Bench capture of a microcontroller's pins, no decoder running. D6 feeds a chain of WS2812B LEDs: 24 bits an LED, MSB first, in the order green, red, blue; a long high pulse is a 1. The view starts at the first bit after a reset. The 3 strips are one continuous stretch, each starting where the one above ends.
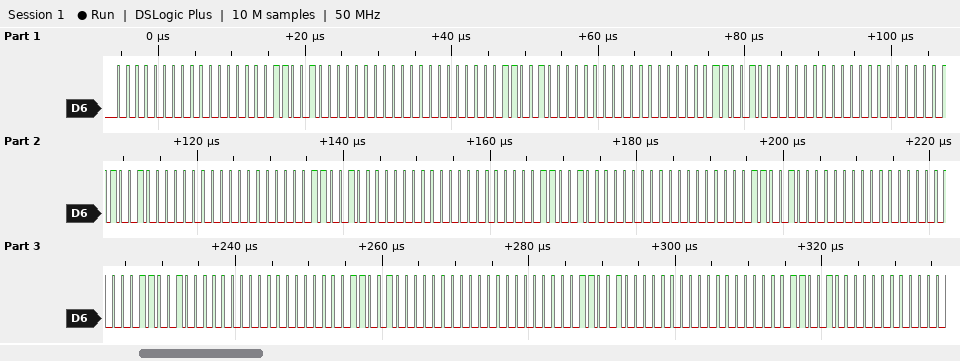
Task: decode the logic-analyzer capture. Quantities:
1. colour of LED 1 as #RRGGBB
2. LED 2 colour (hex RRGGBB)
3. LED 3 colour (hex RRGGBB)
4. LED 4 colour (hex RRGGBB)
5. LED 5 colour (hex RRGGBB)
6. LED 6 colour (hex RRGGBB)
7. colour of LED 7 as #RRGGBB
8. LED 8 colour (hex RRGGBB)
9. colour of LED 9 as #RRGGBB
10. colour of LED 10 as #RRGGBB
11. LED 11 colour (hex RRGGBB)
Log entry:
#000064
#000032
#000064
#000032
#000064
#000032
#000064
#000032
#000064
#000032
#000064
